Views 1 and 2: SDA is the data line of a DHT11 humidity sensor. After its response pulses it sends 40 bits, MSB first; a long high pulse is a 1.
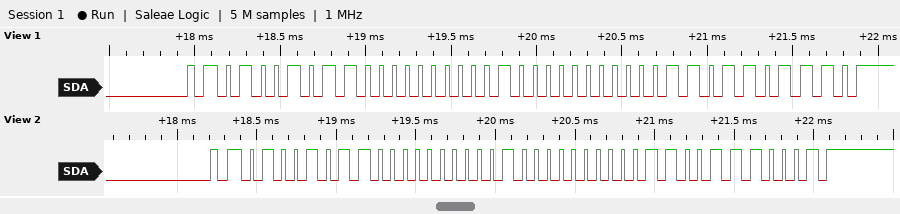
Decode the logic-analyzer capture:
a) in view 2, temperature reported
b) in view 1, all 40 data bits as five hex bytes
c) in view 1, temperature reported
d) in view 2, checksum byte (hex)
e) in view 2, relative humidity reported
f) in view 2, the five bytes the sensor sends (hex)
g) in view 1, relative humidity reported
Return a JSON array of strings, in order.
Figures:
["32.6 °C", "4B 00 20 03 6E", "32.3 °C", "0x71", "75 %", "4B 00 20 06 71", "75 %"]
